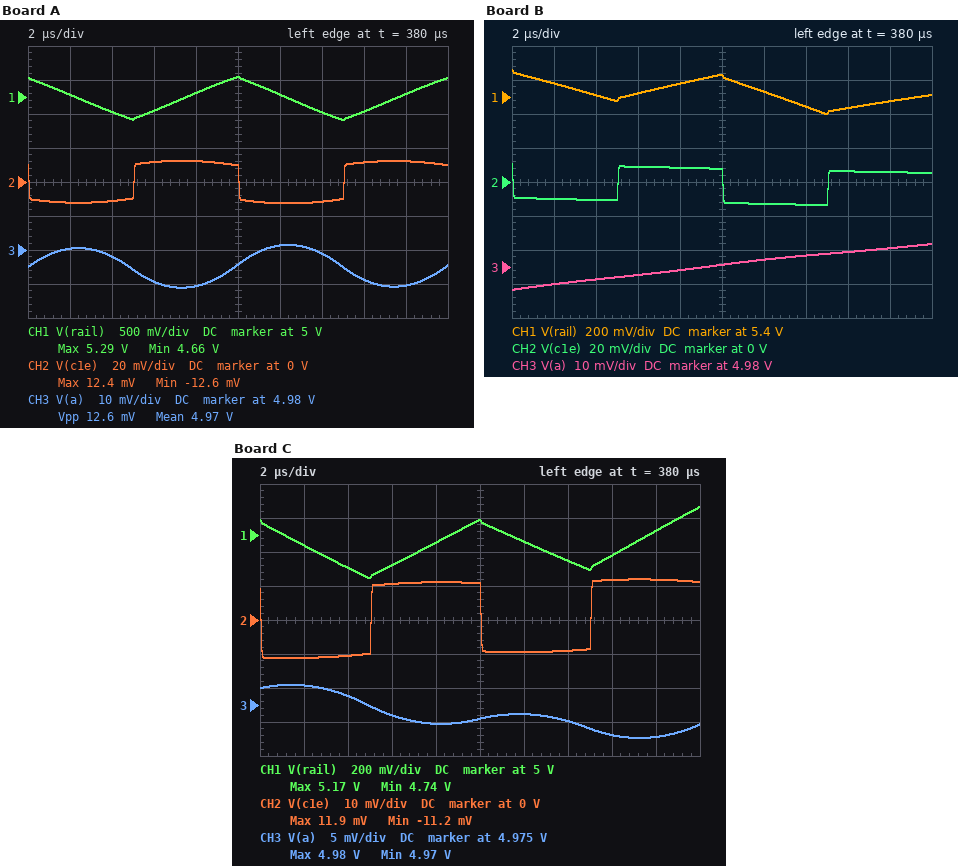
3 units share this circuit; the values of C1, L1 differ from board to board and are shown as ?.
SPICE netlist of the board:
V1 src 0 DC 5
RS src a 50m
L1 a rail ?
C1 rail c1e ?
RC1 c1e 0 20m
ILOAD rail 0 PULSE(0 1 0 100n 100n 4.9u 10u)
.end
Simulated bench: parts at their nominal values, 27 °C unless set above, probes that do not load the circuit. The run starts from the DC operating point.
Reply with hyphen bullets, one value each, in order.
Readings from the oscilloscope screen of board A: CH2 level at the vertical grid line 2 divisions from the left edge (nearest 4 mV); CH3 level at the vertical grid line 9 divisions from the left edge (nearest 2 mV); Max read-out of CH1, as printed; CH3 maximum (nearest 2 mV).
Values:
- -12 mV
- 4.970 V
- 5.29 V
- 4.982 V
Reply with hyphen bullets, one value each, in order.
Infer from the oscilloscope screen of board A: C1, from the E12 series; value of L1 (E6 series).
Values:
- 4.7 µF
- 3.3 µH
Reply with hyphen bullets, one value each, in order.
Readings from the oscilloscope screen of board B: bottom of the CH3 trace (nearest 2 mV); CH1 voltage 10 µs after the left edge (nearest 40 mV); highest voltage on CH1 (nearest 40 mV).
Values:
- 4.974 V
- 5.52 V
- 5.56 V
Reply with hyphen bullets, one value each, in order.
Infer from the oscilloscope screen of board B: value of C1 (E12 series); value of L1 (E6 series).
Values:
- 15 µF
- 33 µH
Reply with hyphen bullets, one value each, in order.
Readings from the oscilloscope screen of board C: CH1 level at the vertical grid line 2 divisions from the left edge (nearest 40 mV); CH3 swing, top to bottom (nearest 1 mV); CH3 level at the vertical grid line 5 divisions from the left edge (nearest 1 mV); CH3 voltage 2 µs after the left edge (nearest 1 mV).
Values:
- 4.80 V
- 8 mV
- 4.973 V
- 4.978 V
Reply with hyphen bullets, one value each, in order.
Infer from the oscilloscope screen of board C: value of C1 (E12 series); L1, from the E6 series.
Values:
- 8.2 µF
- 6.8 µH
